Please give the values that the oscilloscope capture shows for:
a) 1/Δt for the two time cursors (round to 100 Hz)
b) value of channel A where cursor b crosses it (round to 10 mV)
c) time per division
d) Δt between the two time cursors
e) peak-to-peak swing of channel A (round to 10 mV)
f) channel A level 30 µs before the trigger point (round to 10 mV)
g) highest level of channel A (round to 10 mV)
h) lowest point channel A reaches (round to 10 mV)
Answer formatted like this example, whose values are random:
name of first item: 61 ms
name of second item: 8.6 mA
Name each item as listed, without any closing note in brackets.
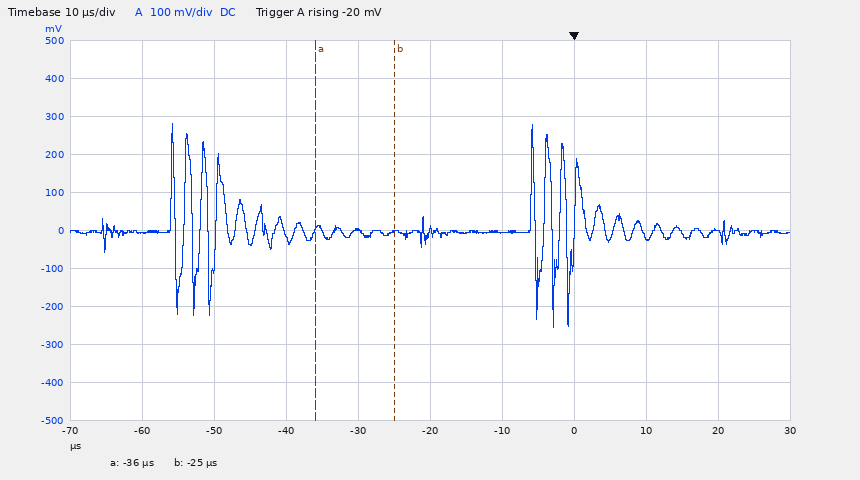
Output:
1/Δt for the two time cursors: 90.9 kHz
value of channel A where cursor b crosses it: 0 mV
time per division: 10 µs
Δt between the two time cursors: 11 µs
peak-to-peak swing of channel A: 540 mV
channel A level 30 µs before the trigger point: 0 mV
highest level of channel A: 280 mV
lowest point channel A reaches: -260 mV
